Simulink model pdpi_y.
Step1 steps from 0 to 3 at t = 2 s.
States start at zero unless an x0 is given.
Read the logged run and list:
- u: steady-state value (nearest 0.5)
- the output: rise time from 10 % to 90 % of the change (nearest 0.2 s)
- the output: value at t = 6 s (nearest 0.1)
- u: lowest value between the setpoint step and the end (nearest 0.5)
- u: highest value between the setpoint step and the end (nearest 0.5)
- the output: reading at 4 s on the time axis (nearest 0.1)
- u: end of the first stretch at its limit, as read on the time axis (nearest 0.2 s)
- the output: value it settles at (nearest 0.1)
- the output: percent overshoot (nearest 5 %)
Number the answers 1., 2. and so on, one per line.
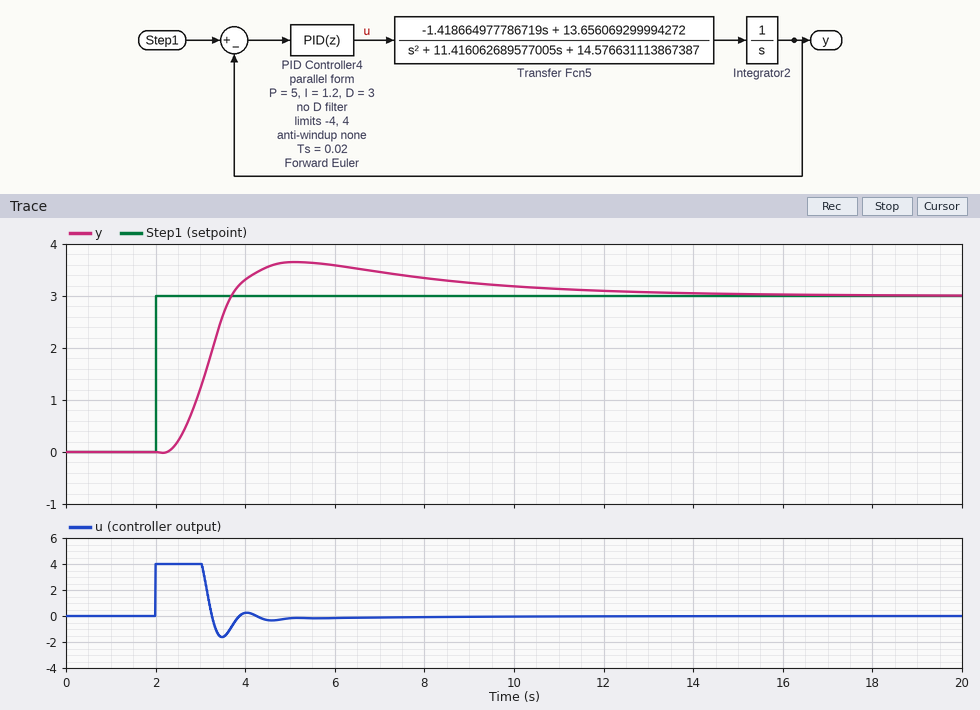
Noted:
1. 0.0
2. 1.0 s
3. 3.6
4. -1.5
5. 4.0
6. 3.3
7. 3.0 s
8. 3.0
9. 20 %
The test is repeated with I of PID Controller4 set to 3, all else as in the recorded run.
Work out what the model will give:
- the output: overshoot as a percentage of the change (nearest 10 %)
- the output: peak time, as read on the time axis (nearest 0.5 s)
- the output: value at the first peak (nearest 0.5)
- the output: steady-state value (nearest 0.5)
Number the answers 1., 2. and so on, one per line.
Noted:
1. 50 %
2. 4.5 s
3. 4.5
4. 3.0
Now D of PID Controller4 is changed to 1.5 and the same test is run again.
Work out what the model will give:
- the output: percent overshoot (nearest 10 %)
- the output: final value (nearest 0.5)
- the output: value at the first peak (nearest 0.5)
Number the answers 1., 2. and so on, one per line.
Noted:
1. 40 %
2. 3.0
3. 4.0
